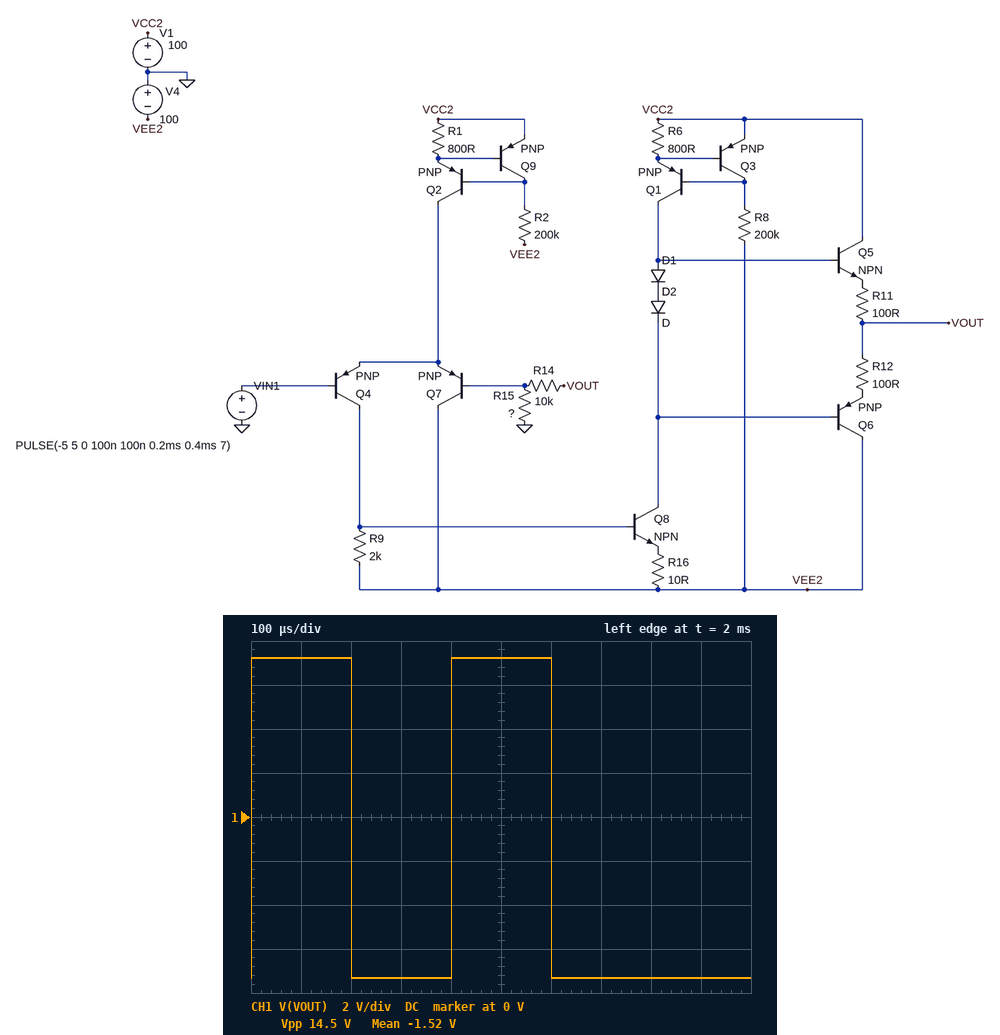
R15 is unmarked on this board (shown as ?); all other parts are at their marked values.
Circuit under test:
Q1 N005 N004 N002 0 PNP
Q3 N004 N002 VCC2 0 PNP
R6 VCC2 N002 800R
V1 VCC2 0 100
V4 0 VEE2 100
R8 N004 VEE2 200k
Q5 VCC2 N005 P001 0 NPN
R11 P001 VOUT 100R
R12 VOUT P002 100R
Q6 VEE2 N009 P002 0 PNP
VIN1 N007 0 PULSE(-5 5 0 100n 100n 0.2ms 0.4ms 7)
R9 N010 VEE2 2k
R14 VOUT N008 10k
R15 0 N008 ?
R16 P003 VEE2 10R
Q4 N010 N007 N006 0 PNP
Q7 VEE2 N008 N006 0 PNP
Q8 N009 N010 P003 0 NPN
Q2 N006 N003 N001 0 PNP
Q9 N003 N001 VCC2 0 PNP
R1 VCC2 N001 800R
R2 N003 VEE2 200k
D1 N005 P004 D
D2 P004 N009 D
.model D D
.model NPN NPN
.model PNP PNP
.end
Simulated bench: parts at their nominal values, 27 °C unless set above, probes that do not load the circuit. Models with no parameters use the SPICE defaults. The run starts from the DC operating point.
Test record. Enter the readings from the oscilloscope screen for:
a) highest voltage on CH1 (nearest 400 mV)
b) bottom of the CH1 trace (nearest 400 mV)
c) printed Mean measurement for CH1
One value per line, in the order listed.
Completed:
7.2 V
-7.2 V
-1.52 V
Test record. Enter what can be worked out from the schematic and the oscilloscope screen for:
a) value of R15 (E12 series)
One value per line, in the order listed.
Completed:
22 kΩ
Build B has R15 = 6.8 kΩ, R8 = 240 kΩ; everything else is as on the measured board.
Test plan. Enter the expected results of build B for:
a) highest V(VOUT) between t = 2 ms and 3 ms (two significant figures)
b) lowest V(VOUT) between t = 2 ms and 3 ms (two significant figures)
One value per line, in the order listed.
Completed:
12 V
-12 V
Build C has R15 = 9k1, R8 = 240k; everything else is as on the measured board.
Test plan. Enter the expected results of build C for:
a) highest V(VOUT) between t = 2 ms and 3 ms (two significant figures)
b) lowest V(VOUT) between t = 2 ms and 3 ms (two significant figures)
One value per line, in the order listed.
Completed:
10 V
-11 V
